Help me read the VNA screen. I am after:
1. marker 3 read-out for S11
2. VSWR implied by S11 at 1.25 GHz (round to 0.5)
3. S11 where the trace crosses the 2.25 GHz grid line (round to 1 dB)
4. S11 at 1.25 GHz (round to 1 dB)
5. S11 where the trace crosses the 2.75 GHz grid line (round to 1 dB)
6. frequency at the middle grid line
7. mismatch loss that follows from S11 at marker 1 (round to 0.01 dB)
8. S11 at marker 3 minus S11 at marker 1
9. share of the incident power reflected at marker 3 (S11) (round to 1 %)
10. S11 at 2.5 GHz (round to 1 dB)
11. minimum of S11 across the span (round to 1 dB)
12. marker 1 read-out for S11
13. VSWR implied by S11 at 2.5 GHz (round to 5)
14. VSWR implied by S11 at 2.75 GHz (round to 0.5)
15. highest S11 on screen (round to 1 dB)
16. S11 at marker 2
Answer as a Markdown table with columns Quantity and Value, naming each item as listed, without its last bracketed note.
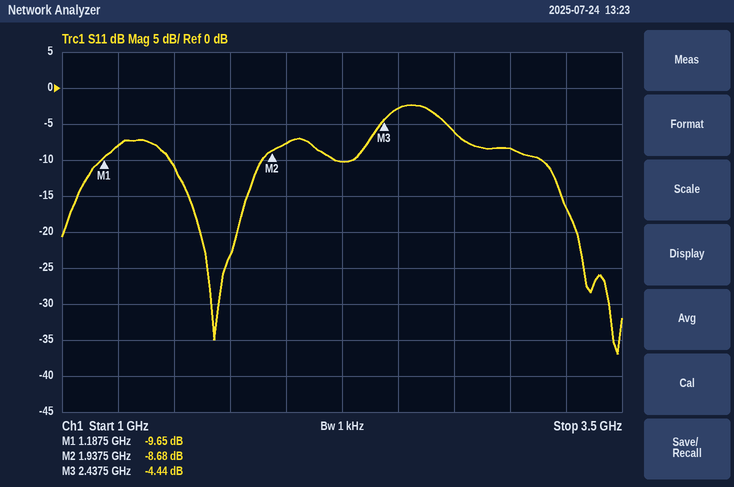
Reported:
| Quantity | Value |
|---|---|
| marker 3 read-out for S11 | -4.44 dB |
| VSWR implied by S11 at 1.25 GHz | 2.5 |
| S11 where the trace crosses the 2.25 GHz grid line | -10 dB |
| S11 at 1.25 GHz | -8 dB |
| S11 where the trace crosses the 2.75 GHz grid line | -6 dB |
| frequency at the middle grid line | 2.25 GHz |
| mismatch loss that follows from S11 at marker 1 | 0.50 dB |
| S11 at marker 3 minus S11 at marker 1 | 5.21 dB |
| share of the incident power reflected at marker 3 (S11) | 36 % |
| S11 at 2.5 GHz | -3 dB |
| minimum of S11 across the span | -37 dB |
| marker 1 read-out for S11 | -9.65 dB |
| VSWR implied by S11 at 2.5 GHz | 5 |
| VSWR implied by S11 at 2.75 GHz | 3.0 |
| highest S11 on screen | -2 dB |
| S11 at marker 2 | -8.68 dB |
